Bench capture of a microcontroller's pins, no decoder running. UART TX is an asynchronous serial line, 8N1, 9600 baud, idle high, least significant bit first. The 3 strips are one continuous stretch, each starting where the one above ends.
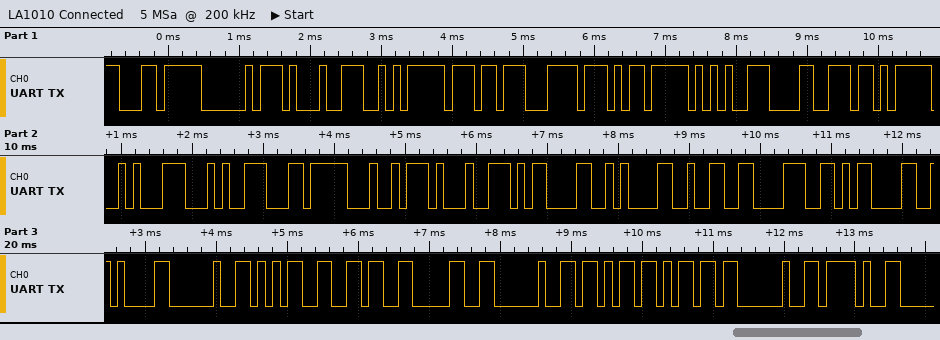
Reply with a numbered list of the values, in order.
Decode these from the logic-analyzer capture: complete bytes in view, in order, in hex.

1. EC A0 91 EA B7 BC ED 95 98 EB 8A 94 EC A4 91 0D 0A 32 38 0D 0A 20 35 36 30 20 6B 6D 20 2F
